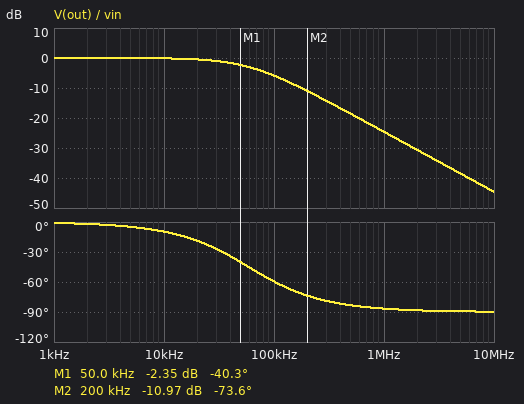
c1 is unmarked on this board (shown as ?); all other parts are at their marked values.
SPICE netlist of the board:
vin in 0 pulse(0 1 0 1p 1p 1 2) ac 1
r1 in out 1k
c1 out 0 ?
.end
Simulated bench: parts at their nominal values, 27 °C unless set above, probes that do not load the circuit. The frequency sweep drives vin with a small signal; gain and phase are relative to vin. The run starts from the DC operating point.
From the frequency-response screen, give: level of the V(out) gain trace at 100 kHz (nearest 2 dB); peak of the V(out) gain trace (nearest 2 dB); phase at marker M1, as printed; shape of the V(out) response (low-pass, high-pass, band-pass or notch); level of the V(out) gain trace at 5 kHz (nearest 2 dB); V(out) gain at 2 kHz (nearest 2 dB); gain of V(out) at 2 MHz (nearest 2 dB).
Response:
-6 dB
0 dB
-40.3 deg
low-pass
0 dB
0 dB
-30 dB
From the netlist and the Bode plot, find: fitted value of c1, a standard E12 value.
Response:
2.7 nF
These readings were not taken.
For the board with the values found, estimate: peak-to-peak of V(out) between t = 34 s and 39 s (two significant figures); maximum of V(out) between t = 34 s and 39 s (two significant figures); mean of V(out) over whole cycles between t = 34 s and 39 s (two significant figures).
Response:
1.0 V
1.0 V
500 mV
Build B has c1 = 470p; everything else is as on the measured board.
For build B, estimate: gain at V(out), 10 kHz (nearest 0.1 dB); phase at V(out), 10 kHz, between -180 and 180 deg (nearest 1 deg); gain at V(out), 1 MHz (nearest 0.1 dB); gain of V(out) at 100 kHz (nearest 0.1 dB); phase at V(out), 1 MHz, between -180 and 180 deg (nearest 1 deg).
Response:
0 dB
-2 deg
-9.9 dB
-0.4 dB
-71 deg
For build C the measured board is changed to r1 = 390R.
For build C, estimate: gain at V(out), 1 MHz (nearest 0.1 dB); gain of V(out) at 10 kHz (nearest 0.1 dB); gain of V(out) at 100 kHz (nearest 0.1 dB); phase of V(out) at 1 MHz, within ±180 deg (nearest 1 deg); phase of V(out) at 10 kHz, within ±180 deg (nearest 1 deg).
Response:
-16.5 dB
0 dB
-1.6 dB
-81 deg
-4 deg
